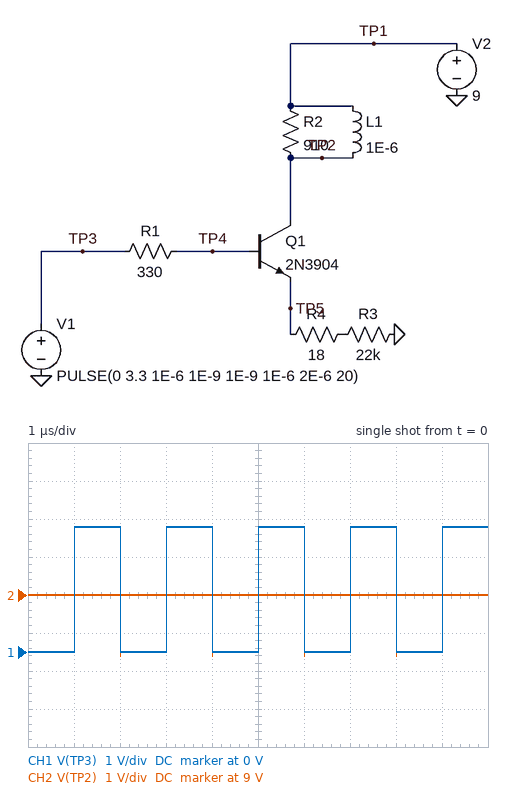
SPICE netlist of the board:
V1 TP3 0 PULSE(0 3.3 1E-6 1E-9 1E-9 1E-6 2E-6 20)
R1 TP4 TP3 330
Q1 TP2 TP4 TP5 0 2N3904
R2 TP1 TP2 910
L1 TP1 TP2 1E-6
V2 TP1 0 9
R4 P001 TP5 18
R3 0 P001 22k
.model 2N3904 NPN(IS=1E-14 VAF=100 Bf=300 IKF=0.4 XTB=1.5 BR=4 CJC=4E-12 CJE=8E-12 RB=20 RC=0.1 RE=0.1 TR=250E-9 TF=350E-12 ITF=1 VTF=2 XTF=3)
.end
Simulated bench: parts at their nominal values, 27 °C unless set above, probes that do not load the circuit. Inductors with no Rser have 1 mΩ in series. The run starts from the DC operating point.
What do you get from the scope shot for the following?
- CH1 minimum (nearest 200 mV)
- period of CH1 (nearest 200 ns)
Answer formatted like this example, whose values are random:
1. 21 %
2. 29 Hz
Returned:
1. 0 V
2. 2.0 µs
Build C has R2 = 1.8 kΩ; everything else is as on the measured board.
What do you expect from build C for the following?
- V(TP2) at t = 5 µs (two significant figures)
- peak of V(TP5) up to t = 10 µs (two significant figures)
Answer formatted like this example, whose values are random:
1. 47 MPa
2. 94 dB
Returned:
1. 9.0 V
2. 3.4 V
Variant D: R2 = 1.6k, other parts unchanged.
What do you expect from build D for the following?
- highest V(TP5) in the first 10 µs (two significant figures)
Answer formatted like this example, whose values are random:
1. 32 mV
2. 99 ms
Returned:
1. 3.4 V
